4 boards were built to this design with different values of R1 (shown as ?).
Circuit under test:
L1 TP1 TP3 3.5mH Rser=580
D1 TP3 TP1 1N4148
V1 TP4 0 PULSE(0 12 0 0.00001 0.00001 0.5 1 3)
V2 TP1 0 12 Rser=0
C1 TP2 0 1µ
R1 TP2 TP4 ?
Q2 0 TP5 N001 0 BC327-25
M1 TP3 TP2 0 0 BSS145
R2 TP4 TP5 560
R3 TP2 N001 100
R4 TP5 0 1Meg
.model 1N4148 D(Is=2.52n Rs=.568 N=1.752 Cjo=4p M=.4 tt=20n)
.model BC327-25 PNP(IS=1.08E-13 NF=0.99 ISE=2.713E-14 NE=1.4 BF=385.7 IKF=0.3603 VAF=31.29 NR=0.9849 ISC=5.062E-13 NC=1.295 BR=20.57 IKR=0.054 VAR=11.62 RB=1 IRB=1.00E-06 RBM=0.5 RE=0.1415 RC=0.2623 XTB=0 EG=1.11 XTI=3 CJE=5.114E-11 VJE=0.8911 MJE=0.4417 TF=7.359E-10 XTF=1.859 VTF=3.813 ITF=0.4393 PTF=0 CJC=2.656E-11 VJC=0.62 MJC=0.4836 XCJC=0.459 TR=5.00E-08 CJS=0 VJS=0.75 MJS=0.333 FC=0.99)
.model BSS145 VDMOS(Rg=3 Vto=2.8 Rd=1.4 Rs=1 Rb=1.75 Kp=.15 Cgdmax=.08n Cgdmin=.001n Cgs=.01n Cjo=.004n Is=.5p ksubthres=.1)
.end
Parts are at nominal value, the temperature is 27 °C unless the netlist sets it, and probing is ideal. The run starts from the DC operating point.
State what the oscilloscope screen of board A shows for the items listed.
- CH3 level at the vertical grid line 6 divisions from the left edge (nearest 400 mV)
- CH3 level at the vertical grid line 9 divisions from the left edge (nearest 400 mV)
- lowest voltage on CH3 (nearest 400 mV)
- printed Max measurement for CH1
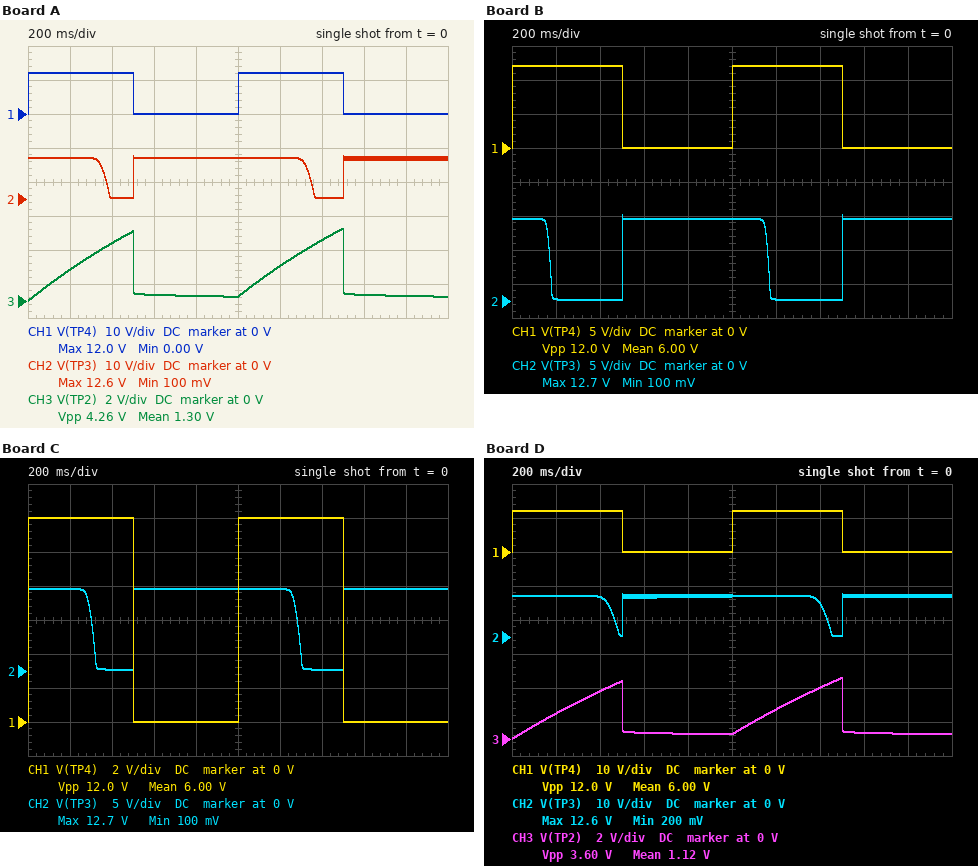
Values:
2.0 V
400 mV
0 V
12.0 V
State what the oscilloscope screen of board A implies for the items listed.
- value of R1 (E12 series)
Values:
1.2 MΩ
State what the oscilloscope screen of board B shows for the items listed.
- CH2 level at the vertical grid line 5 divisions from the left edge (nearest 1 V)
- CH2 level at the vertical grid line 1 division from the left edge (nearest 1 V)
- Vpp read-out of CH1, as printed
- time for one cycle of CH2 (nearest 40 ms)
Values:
12 V
0 V
12.0 V
1.00 s
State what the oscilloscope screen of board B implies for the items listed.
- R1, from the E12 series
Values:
560 kΩ
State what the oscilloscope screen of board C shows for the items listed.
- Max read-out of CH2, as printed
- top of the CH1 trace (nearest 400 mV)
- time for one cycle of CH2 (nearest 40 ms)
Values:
12.7 V
12.0 V
1.00 s
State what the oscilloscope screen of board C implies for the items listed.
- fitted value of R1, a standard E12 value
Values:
1 MΩ
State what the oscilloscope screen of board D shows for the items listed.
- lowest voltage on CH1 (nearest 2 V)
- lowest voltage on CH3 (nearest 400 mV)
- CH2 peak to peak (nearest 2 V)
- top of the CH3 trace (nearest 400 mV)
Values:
0 V
0 V
12 V
3.6 V
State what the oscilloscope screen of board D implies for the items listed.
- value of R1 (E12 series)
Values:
1.5 MΩ
